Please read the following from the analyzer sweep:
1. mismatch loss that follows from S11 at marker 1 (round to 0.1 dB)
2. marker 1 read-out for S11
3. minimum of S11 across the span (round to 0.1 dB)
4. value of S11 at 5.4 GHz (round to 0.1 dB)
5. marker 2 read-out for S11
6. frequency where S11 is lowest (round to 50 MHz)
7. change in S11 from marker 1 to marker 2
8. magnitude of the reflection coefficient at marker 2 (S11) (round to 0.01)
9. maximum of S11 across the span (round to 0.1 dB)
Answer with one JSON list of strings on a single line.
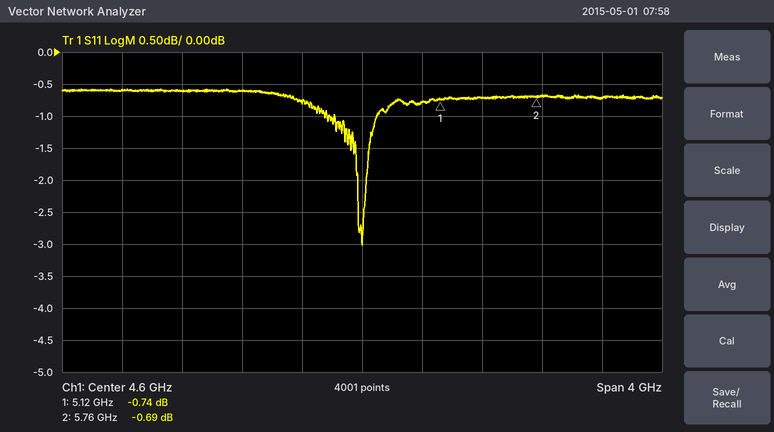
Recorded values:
["8.1 dB", "-0.74 dB", "-3.0 dB", "-0.7 dB", "-0.69 dB", "4.60 GHz", "0.05 dB", "0.92", "-0.6 dB"]
